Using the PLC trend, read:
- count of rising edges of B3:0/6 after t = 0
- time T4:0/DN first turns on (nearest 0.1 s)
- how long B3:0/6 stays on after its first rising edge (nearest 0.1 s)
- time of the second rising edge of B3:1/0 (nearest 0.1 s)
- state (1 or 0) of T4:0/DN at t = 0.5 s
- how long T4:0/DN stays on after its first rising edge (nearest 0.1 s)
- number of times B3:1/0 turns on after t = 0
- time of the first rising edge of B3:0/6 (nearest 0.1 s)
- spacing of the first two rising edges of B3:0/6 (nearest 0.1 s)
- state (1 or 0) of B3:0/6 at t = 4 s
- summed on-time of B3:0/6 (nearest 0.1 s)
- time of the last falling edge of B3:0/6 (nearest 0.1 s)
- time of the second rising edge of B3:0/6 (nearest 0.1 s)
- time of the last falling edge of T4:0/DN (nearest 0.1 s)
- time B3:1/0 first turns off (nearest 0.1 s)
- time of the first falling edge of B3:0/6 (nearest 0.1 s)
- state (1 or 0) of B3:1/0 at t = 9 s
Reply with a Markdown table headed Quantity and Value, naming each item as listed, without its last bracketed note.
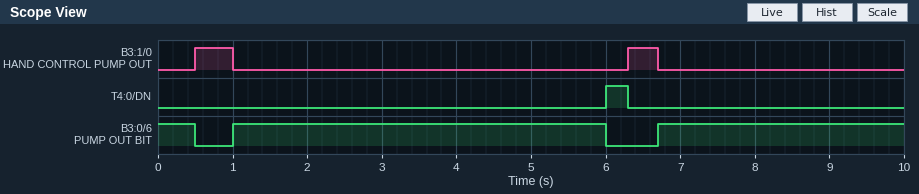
| Quantity | Value |
|---|---|
| count of rising edges of B3:0/6 after t = 0 | 2 |
| time T4:0/DN first turns on | 6.0 s |
| how long B3:0/6 stays on after its first rising edge | 5.0 s |
| time of the second rising edge of B3:1/0 | 6.3 s |
| state (1 or 0) of T4:0/DN at t = 0.5 s | 0 |
| how long T4:0/DN stays on after its first rising edge | 0.3 s |
| number of times B3:1/0 turns on after t = 0 | 2 |
| time of the first rising edge of B3:0/6 | 1.0 s |
| spacing of the first two rising edges of B3:0/6 | 5.7 s |
| state (1 or 0) of B3:0/6 at t = 4 s | 1 |
| summed on-time of B3:0/6 | 8.8 s |
| time of the last falling edge of B3:0/6 | 6.0 s |
| time of the second rising edge of B3:0/6 | 6.7 s |
| time of the last falling edge of T4:0/DN | 6.3 s |
| time B3:1/0 first turns off | 1.0 s |
| time of the first falling edge of B3:0/6 | 0.5 s |
| state (1 or 0) of B3:1/0 at t = 9 s | 0 |
